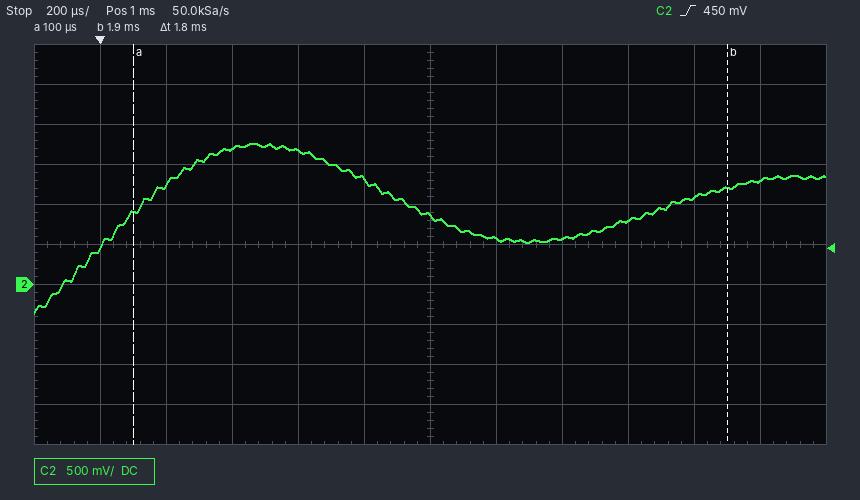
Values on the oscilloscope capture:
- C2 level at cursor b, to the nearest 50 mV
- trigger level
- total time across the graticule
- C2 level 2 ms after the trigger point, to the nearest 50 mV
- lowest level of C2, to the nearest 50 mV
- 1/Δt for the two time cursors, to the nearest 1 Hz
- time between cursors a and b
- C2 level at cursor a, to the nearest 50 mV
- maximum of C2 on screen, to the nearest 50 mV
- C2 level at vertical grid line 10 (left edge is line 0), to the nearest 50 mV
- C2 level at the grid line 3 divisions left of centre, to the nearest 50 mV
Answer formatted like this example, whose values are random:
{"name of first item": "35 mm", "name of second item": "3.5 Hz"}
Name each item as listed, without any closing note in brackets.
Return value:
{"C2 level at cursor b, to the nearest 50 mV": "1.20 V", "trigger level": "450 mV", "total time across the graticule": "2.4 ms", "C2 level 2 ms after the trigger point, to the nearest 50 mV": "1.30 V", "lowest level of C2, to the nearest 50 mV": "-350 mV", "1/Δt for the two time cursors, to the nearest 1 Hz": "556 Hz", "time between cursors a and b": "1.8 ms", "C2 level at cursor a, to the nearest 50 mV": "900 mV", "maximum of C2 on screen, to the nearest 50 mV": "1.75 V", "C2 level at vertical grid line 10 (left edge is line 0), to the nearest 50 mV": "1.10 V", "C2 level at the grid line 3 divisions left of centre, to the nearest 50 mV": "1.70 V"}
